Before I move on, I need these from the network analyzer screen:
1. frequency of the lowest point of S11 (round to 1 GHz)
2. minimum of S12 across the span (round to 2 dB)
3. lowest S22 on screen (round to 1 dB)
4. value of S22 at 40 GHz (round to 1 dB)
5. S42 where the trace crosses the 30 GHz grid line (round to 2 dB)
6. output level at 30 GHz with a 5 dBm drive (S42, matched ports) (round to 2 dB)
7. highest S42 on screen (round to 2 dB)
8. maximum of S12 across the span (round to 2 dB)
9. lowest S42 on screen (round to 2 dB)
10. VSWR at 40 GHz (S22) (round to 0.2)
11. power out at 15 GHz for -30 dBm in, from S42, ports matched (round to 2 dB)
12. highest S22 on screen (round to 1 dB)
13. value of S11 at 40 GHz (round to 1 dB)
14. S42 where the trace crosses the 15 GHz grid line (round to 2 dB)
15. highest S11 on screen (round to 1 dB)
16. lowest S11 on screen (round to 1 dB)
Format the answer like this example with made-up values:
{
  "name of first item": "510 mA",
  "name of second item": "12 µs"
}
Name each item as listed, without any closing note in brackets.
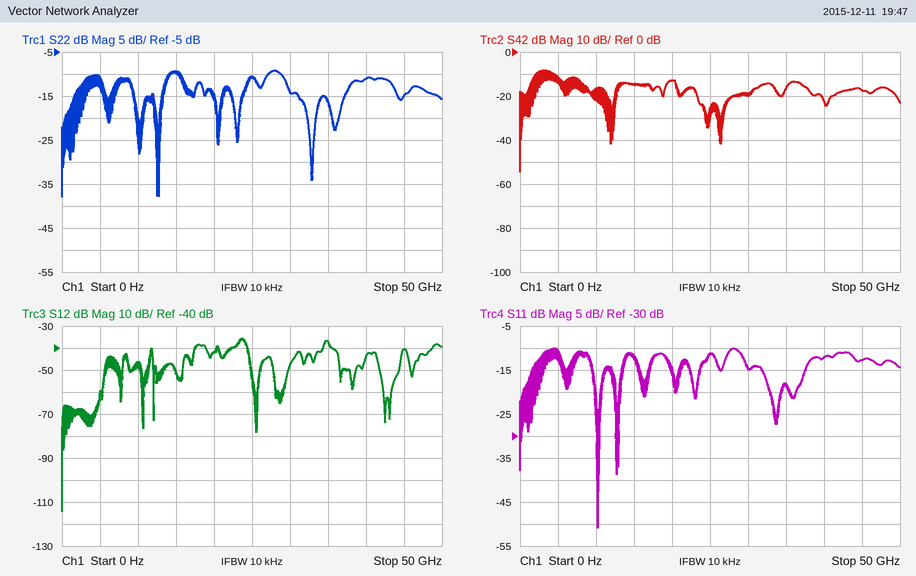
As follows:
{
  "frequency of the lowest point of S11": "10 GHz",
  "minimum of S12 across the span": "-114 dB",
  "lowest S22 on screen": "-38 dB",
  "value of S22 at 40 GHz": "-11 dB",
  "S42 where the trace crosses the 30 GHz grid line": "-20 dB",
  "output level at 30 GHz with a 5 dBm drive (S42, matched ports)": "-14 dBm",
  "highest S42 on screen": "-8 dB",
  "maximum of S12 across the span": "-36 dB",
  "lowest S42 on screen": "-54 dB",
  "VSWR at 40 GHz (S22)": "1.8",
  "power out at 15 GHz for -30 dBm in, from S42, ports matched": "-44 dBm",
  "highest S22 on screen": "-9 dB",
  "value of S11 at 40 GHz": "-12 dB",
  "S42 where the trace crosses the 15 GHz grid line": "-14 dB",
  "highest S11 on screen": "-10 dB",
  "lowest S11 on screen": "-51 dB"
}
